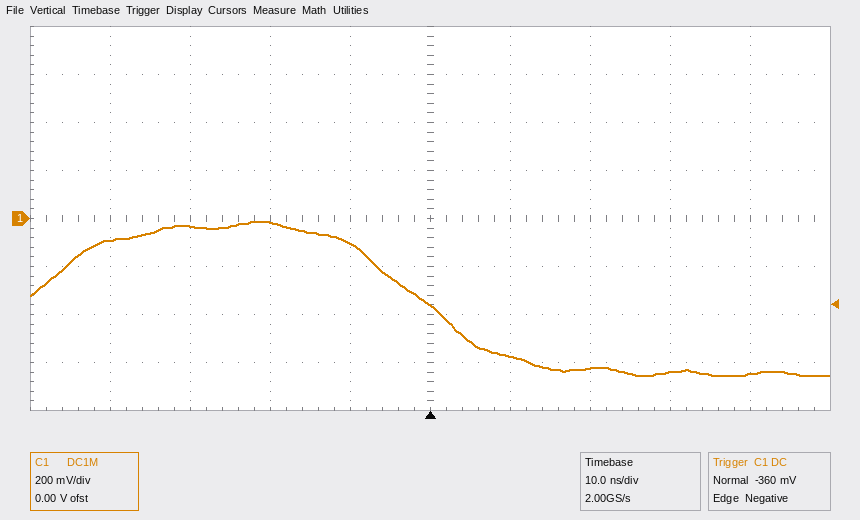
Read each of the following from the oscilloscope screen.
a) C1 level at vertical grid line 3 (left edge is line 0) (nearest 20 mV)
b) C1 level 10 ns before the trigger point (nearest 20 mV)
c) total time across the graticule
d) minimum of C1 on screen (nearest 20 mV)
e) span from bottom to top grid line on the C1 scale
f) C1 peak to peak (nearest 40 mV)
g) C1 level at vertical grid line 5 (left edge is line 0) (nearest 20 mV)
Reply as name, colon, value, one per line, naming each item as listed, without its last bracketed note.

C1 level at vertical grid line 3 (left edge is line 0): -20 mV
C1 level 10 ns before the trigger point: -100 mV
total time across the graticule: 100 ns
minimum of C1 on screen: -660 mV
span from bottom to top grid line on the C1 scale: 1.6 V
C1 peak to peak: 640 mV
C1 level at vertical grid line 5 (left edge is line 0): -360 mV
